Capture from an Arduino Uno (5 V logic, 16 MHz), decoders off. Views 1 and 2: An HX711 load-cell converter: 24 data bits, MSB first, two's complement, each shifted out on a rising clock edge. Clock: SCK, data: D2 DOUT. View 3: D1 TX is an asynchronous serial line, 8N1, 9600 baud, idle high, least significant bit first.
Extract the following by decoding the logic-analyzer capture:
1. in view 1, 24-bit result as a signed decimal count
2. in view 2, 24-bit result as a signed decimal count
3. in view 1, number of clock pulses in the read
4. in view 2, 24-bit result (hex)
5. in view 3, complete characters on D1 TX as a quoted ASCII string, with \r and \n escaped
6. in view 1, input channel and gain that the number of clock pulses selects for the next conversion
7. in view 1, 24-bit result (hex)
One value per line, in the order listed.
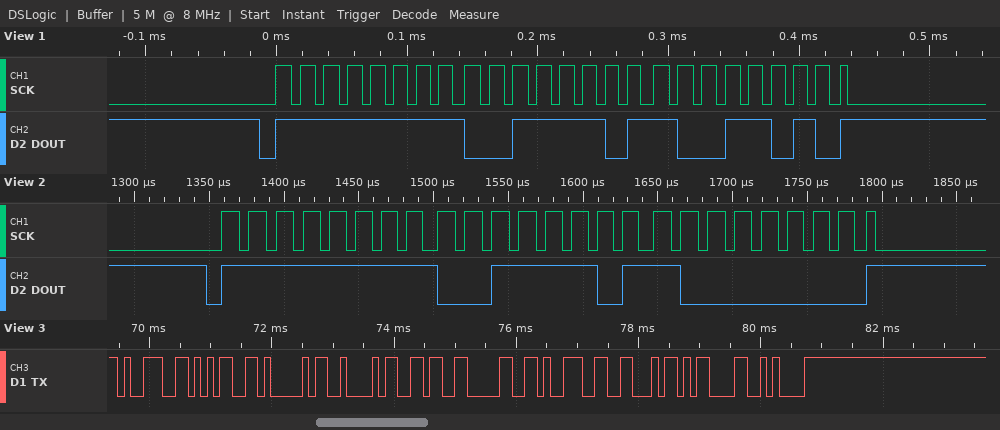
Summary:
-49766
-49792
25
0xFF3D80
"95AB609F\r\n"
channel A, gain 128
0xFF3D9A
